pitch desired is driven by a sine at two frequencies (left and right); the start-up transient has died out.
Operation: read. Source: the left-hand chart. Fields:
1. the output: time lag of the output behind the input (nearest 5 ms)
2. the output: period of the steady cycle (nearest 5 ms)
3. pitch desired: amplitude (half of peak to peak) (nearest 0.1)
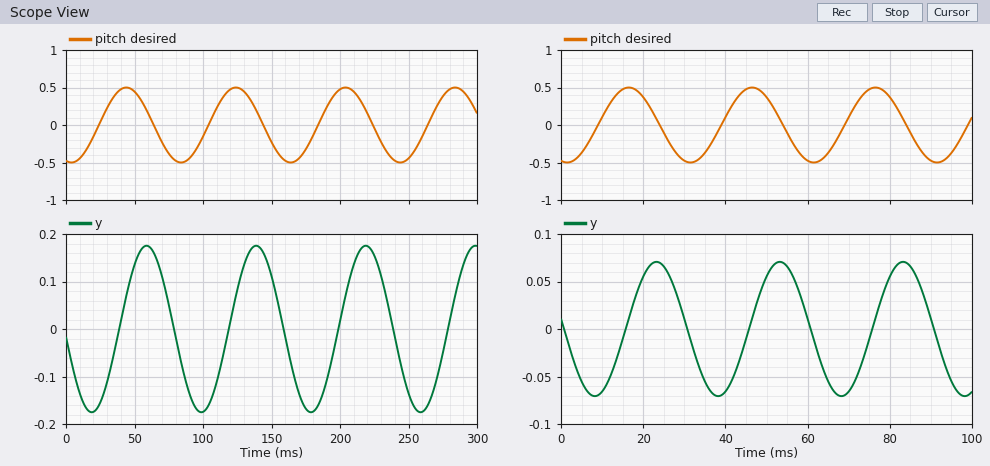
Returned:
15 ms
80 ms
0.5
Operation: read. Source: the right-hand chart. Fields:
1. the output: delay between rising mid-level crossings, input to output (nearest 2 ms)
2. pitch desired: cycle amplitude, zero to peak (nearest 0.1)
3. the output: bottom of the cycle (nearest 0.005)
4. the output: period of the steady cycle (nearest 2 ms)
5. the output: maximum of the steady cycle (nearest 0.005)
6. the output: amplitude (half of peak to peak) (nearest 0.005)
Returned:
6 ms
0.5
-0.070
30 ms
0.070
0.070
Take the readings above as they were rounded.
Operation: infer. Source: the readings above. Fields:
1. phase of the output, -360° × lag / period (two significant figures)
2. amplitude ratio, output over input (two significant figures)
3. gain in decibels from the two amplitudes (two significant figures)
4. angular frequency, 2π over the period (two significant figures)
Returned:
-72°
0.14
-17 dB
0.21 rad/ms
